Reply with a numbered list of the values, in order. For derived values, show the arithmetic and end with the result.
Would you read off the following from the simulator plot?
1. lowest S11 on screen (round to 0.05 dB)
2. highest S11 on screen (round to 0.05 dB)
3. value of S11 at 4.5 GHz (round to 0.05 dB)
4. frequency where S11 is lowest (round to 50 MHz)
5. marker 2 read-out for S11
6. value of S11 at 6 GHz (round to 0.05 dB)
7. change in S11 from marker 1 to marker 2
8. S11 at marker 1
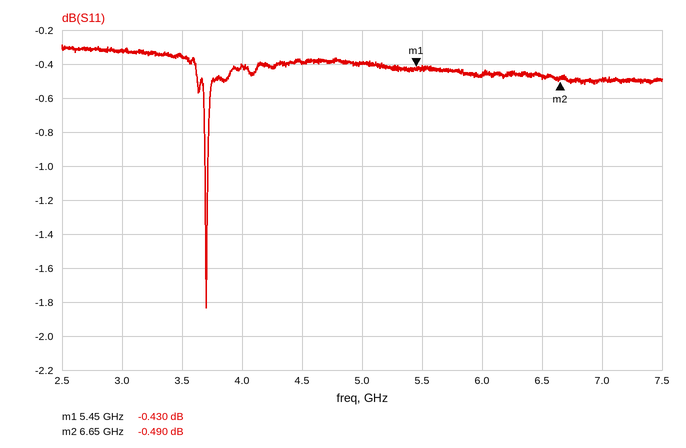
1. -1.85 dB
2. -0.30 dB
3. -0.40 dB
4. 3.70 GHz
5. -0.490 dB
6. -0.45 dB
7. -0.49 − (-0.43) = -0.060 dB
8. -0.430 dB
